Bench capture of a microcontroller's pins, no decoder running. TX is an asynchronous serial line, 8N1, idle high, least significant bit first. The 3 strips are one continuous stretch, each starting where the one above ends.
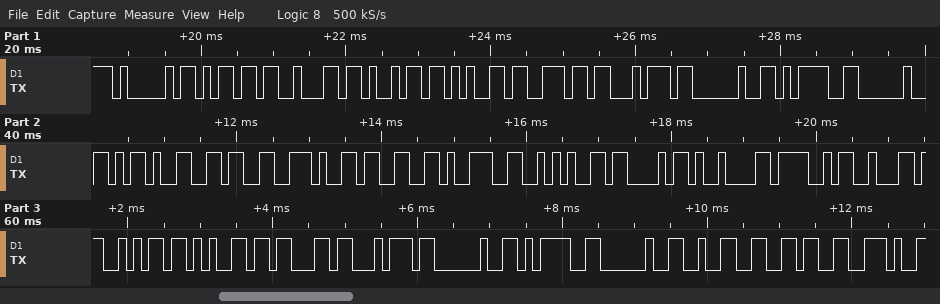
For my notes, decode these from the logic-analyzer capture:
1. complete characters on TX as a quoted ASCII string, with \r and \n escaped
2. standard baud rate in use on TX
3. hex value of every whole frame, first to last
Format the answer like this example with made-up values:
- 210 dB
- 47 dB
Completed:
- "Ambient = -6.39*C\tObject = 26."
- 9600 baud
- 41 6D 62 69 65 6E 74 20 3D 20 2D 36 2E 33 39 2A 43 09 4F 62 6A 65 63 74 20 3D 20 32 36 2E
